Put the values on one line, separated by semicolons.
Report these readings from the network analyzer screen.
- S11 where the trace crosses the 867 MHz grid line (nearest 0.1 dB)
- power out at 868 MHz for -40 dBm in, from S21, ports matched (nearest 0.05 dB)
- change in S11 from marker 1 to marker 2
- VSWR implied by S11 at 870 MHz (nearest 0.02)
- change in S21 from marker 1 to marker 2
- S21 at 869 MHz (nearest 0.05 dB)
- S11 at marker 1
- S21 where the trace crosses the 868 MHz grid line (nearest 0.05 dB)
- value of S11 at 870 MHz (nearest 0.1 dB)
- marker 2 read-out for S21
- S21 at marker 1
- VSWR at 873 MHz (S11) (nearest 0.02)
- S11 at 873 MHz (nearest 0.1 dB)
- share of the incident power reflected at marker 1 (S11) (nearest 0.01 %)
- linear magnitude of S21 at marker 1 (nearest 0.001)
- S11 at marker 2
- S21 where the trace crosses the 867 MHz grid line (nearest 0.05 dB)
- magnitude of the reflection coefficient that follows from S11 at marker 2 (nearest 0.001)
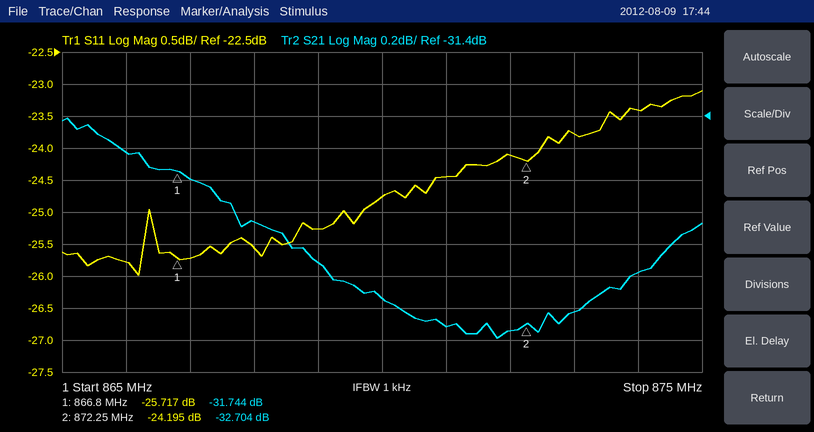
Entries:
-25.7 dB; -72.05 dBm; 1.522 dB; 1.12; -0.960 dB; -32.30 dB; -25.717 dB; -32.05 dB; -24.8 dB; -32.704 dB; -31.744 dB; 1.14; -23.8 dB; 0.27 %; 0.026; -24.195 dB; -31.80 dB; 0.062
